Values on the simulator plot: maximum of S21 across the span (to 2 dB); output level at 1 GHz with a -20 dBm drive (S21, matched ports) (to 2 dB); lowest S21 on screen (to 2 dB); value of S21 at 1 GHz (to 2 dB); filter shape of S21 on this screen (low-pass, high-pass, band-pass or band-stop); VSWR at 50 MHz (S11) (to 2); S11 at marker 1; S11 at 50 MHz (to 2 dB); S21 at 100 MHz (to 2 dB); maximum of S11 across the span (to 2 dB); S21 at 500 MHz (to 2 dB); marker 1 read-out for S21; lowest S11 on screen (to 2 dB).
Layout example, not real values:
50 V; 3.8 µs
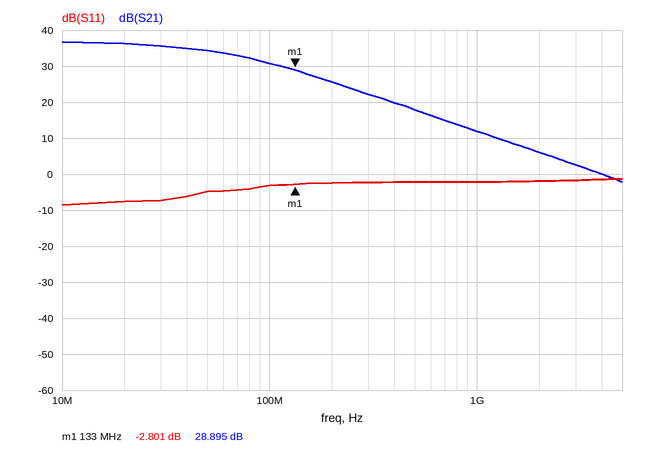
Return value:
36 dB; -8 dBm; -2 dB; 12 dB; low-pass; 4; -2.801 dB; -4 dB; 30 dB; -2 dB; 18 dB; 28.895 dB; -8 dB
